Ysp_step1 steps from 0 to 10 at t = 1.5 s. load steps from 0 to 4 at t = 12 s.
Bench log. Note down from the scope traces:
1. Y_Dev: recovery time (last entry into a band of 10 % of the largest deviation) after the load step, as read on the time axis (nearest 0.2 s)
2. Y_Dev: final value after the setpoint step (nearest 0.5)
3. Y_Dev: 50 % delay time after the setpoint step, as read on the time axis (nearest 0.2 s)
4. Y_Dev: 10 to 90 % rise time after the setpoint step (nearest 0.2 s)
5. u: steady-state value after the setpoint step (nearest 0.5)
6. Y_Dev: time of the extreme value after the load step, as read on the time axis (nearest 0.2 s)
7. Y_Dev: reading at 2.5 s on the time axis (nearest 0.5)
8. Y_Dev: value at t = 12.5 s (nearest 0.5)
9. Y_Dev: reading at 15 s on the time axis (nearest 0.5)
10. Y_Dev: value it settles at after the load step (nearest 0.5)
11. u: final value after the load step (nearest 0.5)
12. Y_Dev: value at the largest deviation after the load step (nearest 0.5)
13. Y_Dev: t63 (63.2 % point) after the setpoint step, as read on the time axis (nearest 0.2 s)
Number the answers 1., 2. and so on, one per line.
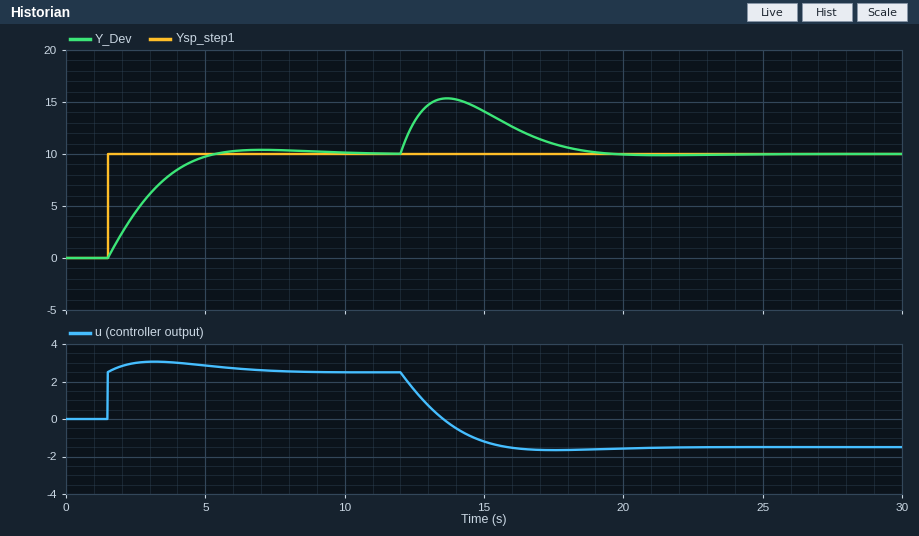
1. 18.2 s
2. 10.0
3. 2.6 s
4. 2.6 s
5. 2.5
6. 13.6 s
7. 4.5
8. 13.0
9. 14.0
10. 10.0
11. -1.5
12. 15.5
13. 3.0 s
